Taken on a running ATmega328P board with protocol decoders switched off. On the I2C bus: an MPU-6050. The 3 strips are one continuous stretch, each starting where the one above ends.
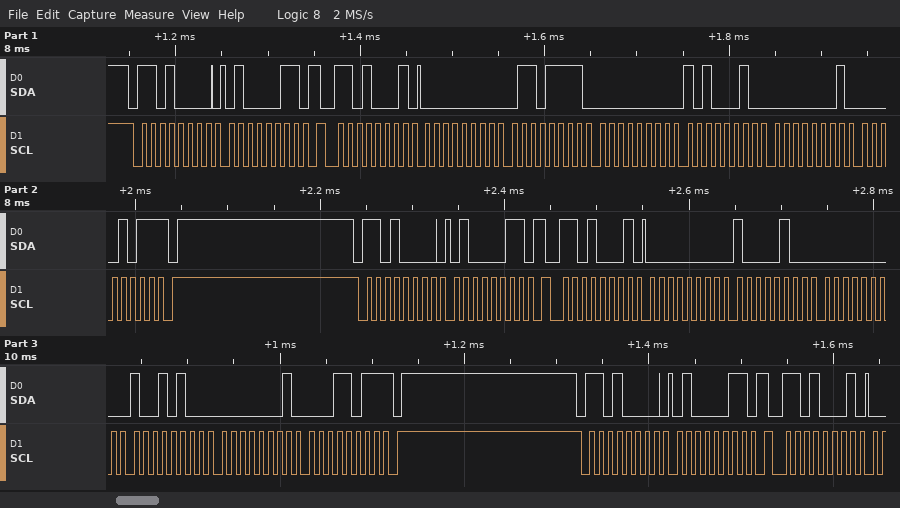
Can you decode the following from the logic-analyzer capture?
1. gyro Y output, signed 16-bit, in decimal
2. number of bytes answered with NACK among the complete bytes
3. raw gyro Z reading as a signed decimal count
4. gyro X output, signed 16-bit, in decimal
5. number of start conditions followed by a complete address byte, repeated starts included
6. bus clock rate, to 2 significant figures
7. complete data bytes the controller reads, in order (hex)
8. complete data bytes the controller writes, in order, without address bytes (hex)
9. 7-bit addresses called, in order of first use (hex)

162
2
267
111
6
100 kHz
00 6F 00 A2 01 0B 00 84 00 94 01 1B
43 43 43
0x68
